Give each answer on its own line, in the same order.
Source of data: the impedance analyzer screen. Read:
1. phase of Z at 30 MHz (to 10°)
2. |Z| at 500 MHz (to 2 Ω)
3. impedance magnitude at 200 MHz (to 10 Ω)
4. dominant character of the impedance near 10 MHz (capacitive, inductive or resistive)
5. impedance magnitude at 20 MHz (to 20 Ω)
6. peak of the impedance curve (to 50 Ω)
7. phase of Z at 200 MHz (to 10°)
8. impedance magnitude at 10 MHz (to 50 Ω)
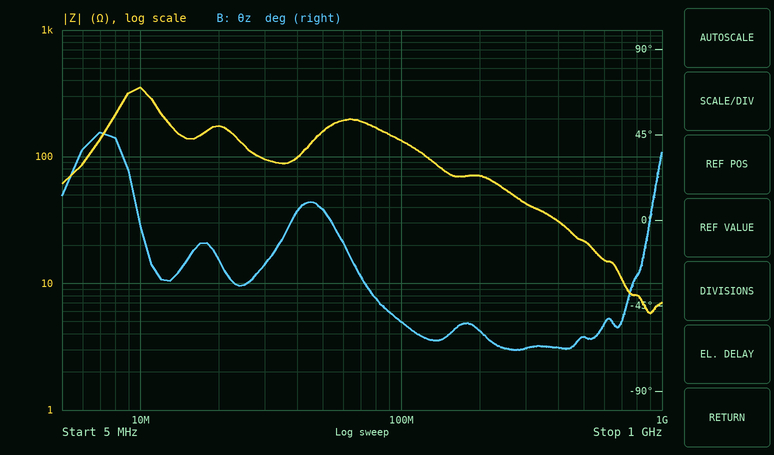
-20°
22 Ω
70 Ω
resistive
180 Ω
350 Ω
-60°
350 Ω
